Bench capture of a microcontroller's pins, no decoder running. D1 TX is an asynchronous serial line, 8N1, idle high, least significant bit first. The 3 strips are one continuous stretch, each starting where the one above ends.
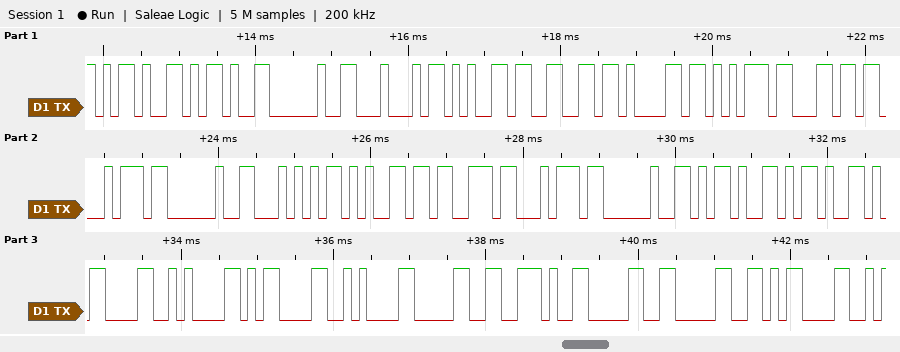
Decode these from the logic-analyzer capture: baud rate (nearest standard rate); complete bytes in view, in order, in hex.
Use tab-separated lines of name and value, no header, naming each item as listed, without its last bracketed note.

baud rate	9600 baud
complete bytes in view, in order, in hex	2D 2D 20 44 65 66 61 75 6C 74 20 54 65 73 74 20 2D 2D 0D 0A 0D 0A 30 2E 30 30 0D
